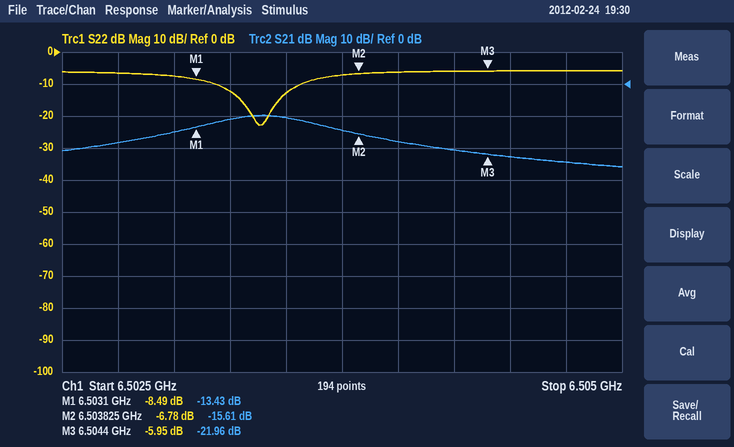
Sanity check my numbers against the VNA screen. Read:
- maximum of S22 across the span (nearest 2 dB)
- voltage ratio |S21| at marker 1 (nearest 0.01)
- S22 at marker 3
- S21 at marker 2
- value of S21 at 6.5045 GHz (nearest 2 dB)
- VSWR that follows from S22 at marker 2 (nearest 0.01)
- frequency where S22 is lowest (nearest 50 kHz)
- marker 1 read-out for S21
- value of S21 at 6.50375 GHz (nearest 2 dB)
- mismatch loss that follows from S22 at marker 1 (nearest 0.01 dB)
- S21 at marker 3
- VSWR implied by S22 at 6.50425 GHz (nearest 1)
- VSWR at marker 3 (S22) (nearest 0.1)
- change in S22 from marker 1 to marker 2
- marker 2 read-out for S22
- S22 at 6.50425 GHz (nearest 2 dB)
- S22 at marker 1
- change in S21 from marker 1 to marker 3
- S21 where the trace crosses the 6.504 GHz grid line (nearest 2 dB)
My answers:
-6 dB
0.21
-5.95 dB
-15.61 dB
-22 dB
2.69
6.50340 GHz
-13.43 dB
-14 dB
0.66 dB
-21.96 dB
3
3.0
1.71 dB
-6.78 dB
-6 dB
-8.49 dB
-8.53 dB
-18 dB
